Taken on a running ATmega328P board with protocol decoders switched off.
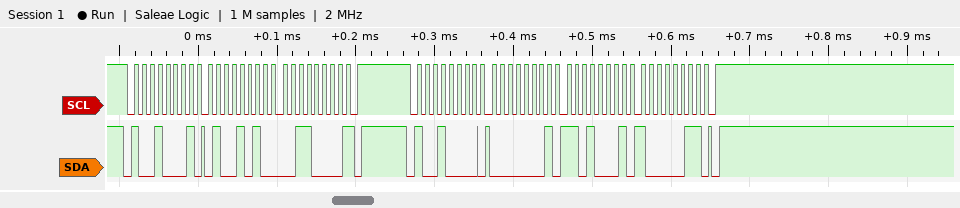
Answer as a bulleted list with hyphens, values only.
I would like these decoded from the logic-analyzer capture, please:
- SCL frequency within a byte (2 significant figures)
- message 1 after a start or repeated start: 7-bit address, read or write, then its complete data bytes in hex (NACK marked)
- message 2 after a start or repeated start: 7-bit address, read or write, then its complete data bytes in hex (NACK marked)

- 100 kHz
- 0x48 read: 4A 30 NACK
- 0x48 write: 01 D1 83
